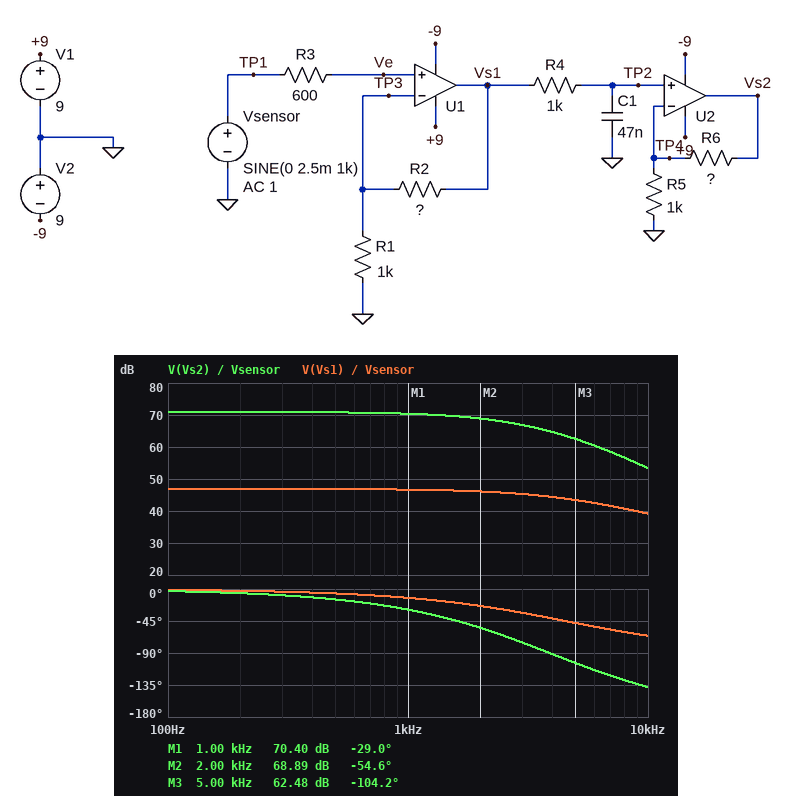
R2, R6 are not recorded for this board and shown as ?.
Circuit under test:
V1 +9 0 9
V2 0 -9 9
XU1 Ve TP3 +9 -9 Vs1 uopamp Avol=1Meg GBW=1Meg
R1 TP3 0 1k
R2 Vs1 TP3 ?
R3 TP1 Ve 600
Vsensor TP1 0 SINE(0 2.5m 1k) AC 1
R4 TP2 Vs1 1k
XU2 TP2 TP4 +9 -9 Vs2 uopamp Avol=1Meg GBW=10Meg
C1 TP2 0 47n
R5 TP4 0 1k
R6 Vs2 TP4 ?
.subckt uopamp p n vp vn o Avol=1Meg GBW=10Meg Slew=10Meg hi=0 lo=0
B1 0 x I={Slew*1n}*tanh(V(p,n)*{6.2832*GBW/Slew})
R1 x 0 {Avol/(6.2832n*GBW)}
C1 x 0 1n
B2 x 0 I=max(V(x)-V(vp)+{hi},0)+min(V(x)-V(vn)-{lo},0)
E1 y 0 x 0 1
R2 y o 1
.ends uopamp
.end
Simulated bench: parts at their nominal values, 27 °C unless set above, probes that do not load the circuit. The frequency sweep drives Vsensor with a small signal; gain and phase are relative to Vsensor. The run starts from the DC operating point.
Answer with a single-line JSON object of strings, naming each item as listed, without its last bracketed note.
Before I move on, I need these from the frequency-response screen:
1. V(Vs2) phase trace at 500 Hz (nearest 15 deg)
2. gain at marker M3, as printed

{"V(Vs2) phase trace at 500 Hz": "-15 deg", "gain at marker M3, as printed": "62.48 dB"}
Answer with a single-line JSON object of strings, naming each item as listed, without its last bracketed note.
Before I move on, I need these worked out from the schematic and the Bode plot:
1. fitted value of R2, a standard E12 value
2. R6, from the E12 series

{"fitted value of R2, a standard E12 value": "220 kΩ", "R6, from the E12 series": "15 kΩ"}
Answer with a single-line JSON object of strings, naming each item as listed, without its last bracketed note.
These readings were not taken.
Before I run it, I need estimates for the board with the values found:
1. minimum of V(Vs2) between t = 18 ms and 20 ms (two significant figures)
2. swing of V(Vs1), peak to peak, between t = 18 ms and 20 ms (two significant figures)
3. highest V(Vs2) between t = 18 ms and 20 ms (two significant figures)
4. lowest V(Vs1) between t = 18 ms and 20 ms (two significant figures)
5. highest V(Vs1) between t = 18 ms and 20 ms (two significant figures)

{"minimum of V(Vs2) between t = 18 ms and 20 ms": "-8.3 V", "swing of V(Vs1), peak to peak, between t = 18 ms and 20 ms": "1.1 V", "highest V(Vs2) between t = 18 ms and 20 ms": "8.3 V", "lowest V(Vs1) between t = 18 ms and 20 ms": "-540 mV", "highest V(Vs1) between t = 18 ms and 20 ms": "540 mV"}
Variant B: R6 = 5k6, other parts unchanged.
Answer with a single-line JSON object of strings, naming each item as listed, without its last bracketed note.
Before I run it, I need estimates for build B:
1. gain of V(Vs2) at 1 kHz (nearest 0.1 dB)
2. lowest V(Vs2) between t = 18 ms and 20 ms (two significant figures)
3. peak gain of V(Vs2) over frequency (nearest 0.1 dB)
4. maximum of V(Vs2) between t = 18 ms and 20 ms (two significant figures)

{"gain of V(Vs2) at 1 kHz": "62.7 dB", "lowest V(Vs2) between t = 18 ms and 20 ms": "-3.4 V", "peak gain of V(Vs2) over frequency": "63.3 dB", "maximum of V(Vs2) between t = 18 ms and 20 ms": "3.4 V"}
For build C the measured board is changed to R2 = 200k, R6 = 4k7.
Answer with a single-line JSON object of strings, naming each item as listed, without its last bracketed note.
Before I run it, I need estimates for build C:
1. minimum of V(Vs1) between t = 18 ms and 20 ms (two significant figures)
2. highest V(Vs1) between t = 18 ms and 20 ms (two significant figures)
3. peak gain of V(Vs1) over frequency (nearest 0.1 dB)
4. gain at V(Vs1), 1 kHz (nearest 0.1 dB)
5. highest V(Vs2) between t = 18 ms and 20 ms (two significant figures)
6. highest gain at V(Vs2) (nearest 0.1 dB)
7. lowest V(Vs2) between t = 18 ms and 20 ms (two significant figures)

{"minimum of V(Vs1) between t = 18 ms and 20 ms": "-490 mV", "highest V(Vs1) between t = 18 ms and 20 ms": "490 mV", "peak gain of V(Vs1) over frequency": "46.1 dB", "gain at V(Vs1), 1 kHz": "45.9 dB", "highest V(Vs2) between t = 18 ms and 20 ms": "2.7 V", "highest gain at V(Vs2)": "61.2 dB", "lowest V(Vs2) between t = 18 ms and 20 ms": "-2.7 V"}
